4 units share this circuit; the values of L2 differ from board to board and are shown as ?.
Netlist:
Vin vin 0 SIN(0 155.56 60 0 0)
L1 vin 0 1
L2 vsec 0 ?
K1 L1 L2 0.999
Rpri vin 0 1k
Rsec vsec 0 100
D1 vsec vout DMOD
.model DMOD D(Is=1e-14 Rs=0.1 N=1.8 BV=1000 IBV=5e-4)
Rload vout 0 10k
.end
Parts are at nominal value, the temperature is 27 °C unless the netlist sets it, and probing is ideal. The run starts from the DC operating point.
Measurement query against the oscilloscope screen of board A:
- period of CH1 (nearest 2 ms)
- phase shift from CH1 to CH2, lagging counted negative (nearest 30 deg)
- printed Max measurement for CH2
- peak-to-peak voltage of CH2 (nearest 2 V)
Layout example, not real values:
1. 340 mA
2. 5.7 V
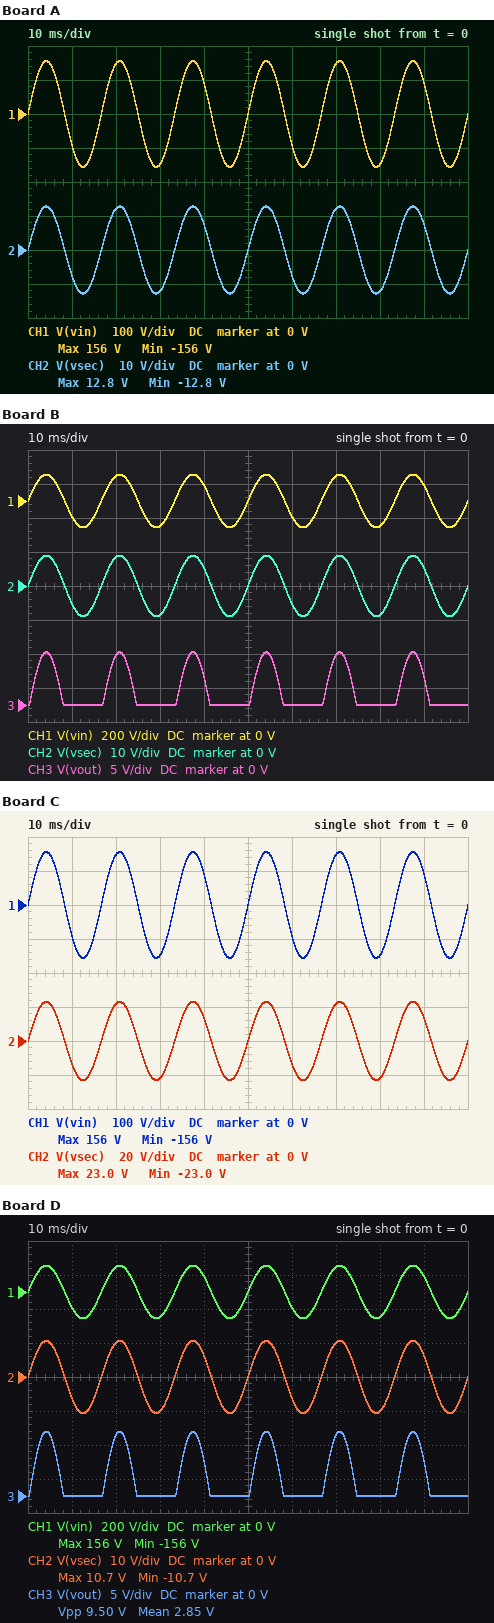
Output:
1. 16 ms
2. 0 deg
3. 12.8 V
4. 26 V
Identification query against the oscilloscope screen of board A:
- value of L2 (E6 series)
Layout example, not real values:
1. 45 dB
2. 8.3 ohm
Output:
1. 6.8 mH
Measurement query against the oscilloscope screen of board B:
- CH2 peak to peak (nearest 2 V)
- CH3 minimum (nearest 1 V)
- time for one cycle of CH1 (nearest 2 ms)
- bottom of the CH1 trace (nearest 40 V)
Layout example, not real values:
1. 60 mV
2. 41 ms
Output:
1. 18 V
2. 0 V
3. 16 ms
4. -160 V
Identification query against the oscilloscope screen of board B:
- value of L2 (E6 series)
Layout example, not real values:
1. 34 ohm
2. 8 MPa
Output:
1. 3.3 mH
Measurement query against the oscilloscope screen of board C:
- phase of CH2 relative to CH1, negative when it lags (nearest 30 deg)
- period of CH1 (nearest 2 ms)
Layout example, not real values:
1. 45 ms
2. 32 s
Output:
1. 0 deg
2. 16 ms
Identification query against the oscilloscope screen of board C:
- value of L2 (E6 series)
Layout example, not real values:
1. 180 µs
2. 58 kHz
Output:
1. 22 mH
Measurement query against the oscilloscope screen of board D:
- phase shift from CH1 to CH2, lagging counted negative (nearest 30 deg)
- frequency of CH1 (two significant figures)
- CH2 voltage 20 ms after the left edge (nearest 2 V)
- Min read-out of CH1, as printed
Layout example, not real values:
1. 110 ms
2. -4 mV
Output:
1. 0 deg
2. 60 Hz
3. 10 V
4. -156 V
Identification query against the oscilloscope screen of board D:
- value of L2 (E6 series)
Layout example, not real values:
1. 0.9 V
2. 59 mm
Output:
1. 4.7 mH
